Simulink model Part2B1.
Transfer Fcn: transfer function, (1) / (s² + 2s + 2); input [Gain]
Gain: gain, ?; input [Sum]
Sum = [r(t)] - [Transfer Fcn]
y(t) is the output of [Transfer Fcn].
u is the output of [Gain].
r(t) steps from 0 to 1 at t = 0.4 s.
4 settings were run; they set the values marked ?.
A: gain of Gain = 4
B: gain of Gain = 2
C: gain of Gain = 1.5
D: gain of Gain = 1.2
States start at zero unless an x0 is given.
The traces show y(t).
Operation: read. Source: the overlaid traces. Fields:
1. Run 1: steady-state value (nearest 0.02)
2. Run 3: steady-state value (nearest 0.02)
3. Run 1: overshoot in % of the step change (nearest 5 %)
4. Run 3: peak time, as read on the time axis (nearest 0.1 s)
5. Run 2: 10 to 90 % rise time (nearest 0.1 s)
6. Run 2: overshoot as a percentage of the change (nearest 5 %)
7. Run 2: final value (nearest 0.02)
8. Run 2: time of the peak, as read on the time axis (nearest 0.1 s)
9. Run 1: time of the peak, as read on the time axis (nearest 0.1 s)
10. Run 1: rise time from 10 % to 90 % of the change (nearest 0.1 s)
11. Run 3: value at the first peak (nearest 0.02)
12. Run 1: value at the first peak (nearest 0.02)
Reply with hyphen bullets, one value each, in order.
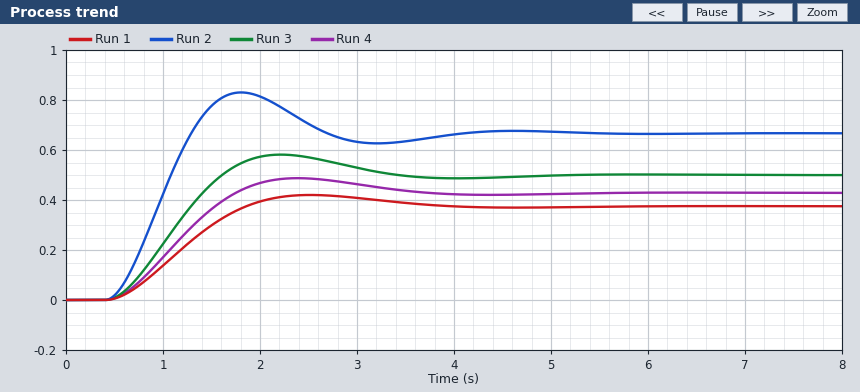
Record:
- 0.38
- 0.50
- 10 %
- 2.2 s
- 0.6 s
- 25 %
- 0.66
- 1.8 s
- 2.5 s
- 1.0 s
- 0.58
- 0.42
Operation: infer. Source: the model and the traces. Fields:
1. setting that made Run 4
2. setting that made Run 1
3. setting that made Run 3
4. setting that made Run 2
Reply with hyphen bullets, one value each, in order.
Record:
- C
- D
- B
- A
